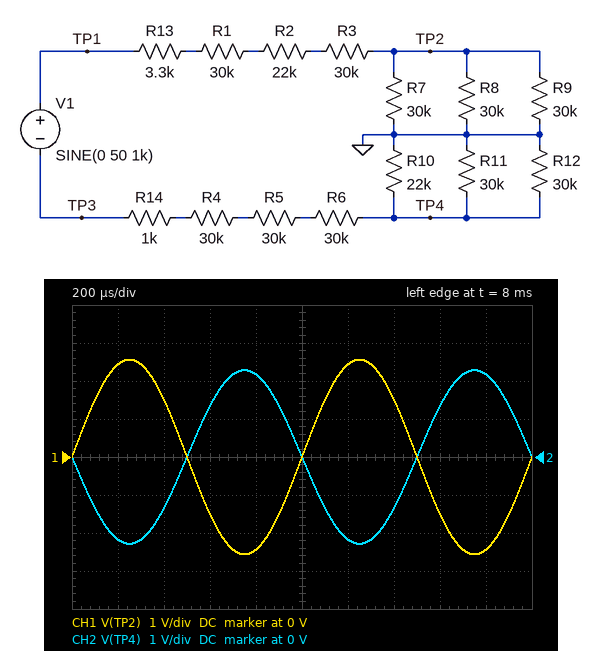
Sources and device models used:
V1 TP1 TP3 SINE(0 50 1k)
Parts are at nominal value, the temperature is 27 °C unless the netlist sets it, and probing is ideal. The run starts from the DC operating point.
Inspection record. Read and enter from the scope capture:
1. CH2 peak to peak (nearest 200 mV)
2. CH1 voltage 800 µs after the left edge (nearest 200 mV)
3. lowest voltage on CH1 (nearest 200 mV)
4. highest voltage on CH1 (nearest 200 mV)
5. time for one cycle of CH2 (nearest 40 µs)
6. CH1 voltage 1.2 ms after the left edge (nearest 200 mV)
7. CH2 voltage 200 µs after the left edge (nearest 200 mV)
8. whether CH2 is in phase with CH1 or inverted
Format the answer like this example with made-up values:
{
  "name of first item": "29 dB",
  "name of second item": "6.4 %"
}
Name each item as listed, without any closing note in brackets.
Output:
{
  "CH2 peak to peak": "4.6 V",
  "CH1 voltage 800 µs after the left edge": "-2.4 V",
  "lowest voltage on CH1": "-2.6 V",
  "highest voltage on CH1": "2.6 V",
  "time for one cycle of CH2": "1.00 ms",
  "CH1 voltage 1.2 ms after the left edge": "2.4 V",
  "CH2 voltage 200 µs after the left edge": "-2.2 V",
  "whether CH2 is in phase with CH1 or inverted": "inverted"
}
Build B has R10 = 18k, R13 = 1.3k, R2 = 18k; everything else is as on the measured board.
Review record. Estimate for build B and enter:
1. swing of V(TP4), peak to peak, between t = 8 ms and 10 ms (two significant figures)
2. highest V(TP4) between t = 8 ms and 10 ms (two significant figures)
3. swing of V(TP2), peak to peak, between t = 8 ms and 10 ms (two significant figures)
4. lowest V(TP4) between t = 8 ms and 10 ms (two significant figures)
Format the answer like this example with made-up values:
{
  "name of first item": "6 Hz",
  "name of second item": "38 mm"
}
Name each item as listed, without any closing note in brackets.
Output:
{
  "swing of V(TP4), peak to peak, between t = 8 ms and 10 ms": "4.3 V",
  "highest V(TP4) between t = 8 ms and 10 ms": "2.2 V",
  "swing of V(TP2), peak to peak, between t = 8 ms and 10 ms": "5.3 V",
  "lowest V(TP4) between t = 8 ms and 10 ms": "-2.2 V"
}
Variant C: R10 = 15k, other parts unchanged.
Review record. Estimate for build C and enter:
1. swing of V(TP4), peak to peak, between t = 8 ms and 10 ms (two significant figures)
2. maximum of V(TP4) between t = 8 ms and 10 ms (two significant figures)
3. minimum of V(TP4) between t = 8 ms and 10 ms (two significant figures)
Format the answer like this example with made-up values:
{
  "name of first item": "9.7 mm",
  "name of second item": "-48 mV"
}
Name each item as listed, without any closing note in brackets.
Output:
{
  "swing of V(TP4), peak to peak, between t = 8 ms and 10 ms": "3.9 V",
  "maximum of V(TP4) between t = 8 ms and 10 ms": "1.9 V",
  "minimum of V(TP4) between t = 8 ms and 10 ms": "-1.9 V"
}
